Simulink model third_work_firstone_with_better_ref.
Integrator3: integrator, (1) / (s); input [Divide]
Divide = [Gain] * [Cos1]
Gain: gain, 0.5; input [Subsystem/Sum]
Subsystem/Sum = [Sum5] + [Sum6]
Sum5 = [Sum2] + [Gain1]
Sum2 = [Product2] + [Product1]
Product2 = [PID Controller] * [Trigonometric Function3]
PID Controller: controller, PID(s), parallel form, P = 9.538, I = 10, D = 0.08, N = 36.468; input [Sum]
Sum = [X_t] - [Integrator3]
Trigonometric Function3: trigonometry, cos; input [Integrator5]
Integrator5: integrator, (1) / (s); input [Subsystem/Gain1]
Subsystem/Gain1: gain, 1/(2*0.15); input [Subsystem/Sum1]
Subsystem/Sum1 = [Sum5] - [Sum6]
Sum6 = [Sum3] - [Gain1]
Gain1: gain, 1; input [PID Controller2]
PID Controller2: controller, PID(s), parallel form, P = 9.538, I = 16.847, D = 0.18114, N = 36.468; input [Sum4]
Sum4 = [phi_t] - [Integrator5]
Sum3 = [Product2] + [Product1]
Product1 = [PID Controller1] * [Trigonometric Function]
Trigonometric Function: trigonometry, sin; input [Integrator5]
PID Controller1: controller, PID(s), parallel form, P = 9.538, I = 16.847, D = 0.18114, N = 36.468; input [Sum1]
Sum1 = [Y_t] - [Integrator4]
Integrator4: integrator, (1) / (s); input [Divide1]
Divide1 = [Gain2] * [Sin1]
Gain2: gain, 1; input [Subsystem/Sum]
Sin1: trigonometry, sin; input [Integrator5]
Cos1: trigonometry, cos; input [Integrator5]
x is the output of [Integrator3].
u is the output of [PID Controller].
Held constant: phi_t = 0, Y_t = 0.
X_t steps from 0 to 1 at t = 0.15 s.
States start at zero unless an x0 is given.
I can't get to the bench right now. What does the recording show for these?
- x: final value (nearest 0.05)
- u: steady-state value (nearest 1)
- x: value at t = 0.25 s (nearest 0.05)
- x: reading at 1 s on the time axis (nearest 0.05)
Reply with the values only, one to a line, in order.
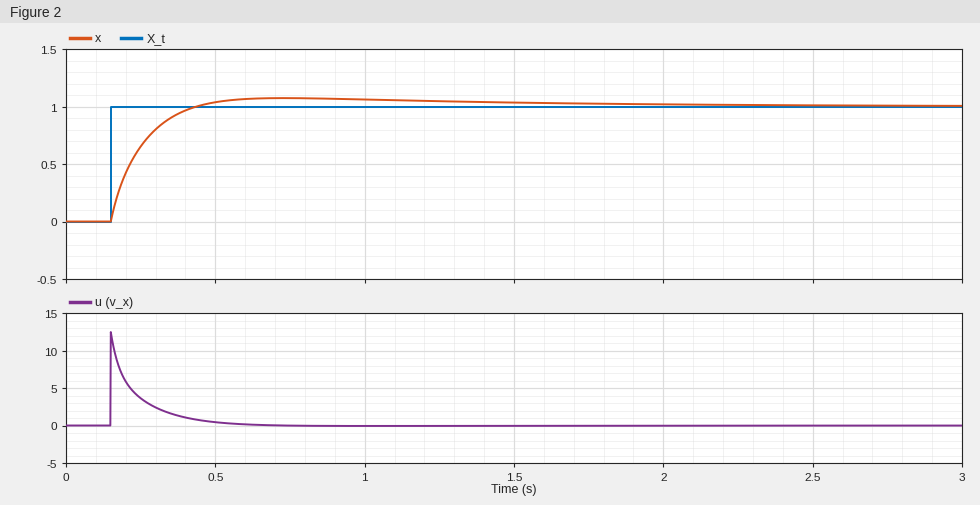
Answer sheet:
1.00
0
0.65
1.05
